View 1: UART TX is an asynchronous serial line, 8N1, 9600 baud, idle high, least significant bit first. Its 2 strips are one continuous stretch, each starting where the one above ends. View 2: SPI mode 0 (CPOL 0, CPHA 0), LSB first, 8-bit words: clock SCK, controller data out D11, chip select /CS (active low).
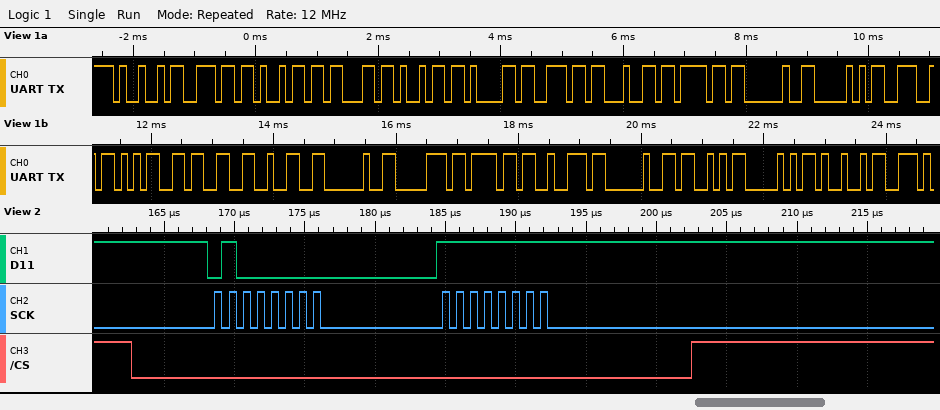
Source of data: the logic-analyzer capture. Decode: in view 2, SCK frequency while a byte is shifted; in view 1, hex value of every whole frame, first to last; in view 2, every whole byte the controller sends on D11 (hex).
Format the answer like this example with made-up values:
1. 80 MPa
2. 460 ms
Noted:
1. 1 MHz
2. 49 6E 69 63 69 61 6E 64 6F 20 50 4E 35 33 32 20 70 6F 72 20 53 50 49
3. 02 FF
